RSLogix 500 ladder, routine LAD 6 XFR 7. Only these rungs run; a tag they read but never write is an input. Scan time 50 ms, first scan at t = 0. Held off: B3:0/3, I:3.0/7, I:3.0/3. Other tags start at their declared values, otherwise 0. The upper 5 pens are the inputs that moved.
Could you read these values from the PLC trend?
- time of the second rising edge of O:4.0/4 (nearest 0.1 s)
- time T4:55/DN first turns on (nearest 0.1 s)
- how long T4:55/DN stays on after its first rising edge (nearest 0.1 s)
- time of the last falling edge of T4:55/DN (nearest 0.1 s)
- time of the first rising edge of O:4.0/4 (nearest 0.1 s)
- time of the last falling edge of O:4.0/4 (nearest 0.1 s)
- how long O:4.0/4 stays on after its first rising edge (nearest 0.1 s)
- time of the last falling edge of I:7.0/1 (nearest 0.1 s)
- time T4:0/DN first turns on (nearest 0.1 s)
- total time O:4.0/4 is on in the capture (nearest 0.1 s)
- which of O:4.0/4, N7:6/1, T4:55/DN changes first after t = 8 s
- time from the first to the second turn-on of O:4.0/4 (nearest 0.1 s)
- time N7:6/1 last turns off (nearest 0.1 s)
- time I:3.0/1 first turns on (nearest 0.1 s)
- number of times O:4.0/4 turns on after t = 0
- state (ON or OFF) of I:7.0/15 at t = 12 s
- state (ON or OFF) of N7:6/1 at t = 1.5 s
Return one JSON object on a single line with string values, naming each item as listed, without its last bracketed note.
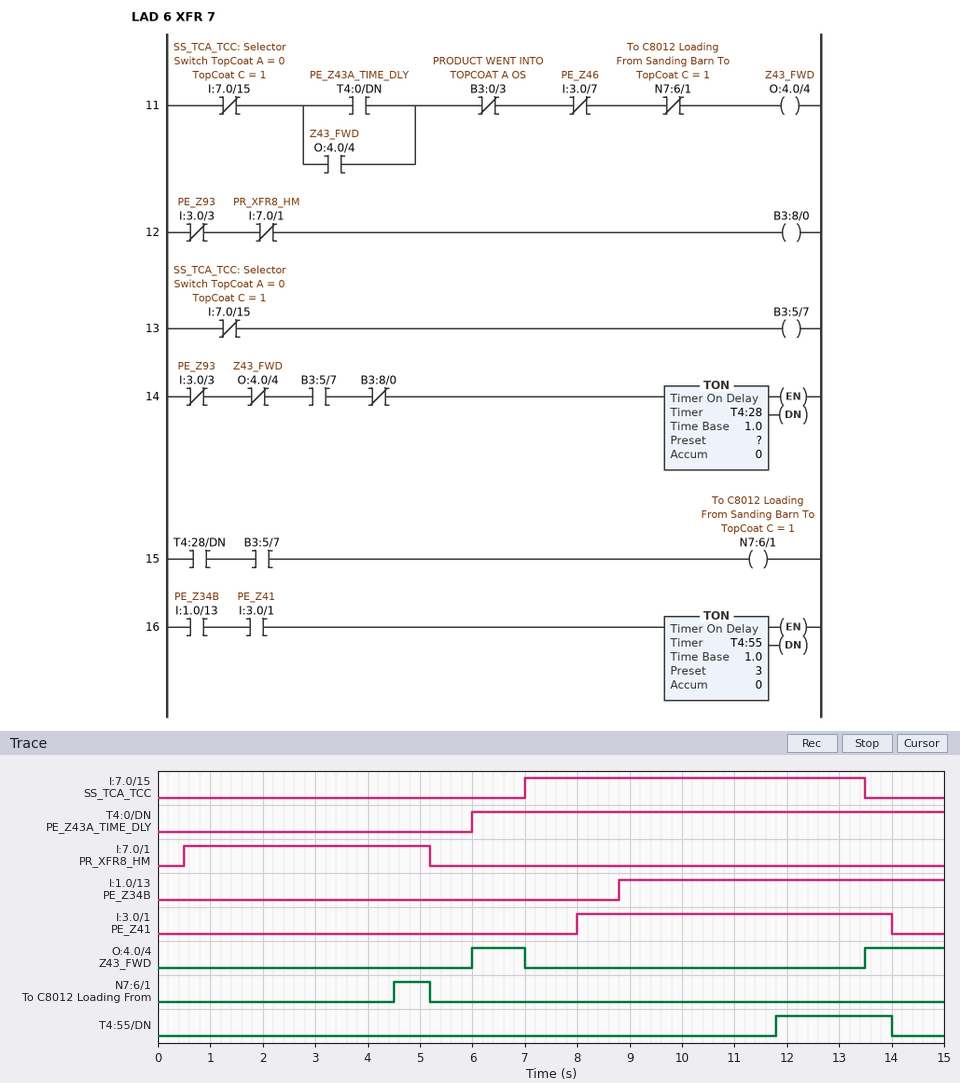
{"time of the second rising edge of O:4.0/4": "13.5 s", "time T4:55/DN first turns on": "11.8 s", "how long T4:55/DN stays on after its first rising edge": "2.2 s", "time of the last falling edge of T4:55/DN": "14.0 s", "time of the first rising edge of O:4.0/4": "6.0 s", "time of the last falling edge of O:4.0/4": "7.0 s", "how long O:4.0/4 stays on after its first rising edge": "1.0 s", "time of the last falling edge of I:7.0/1": "5.2 s", "time T4:0/DN first turns on": "6.0 s", "total time O:4.0/4 is on in the capture": "2.5 s", "which of O:4.0/4, N7:6/1, T4:55/DN changes first after t = 8 s": "T4:55/DN", "time from the first to the second turn-on of O:4.0/4": "7.5 s", "time N7:6/1 last turns off": "5.2 s", "time I:3.0/1 first turns on": "8.0 s", "number of times O:4.0/4 turns on after t = 0": "2", "state (ON or OFF) of I:7.0/15 at t = 12 s": "ON", "state (ON or OFF) of N7:6/1 at t = 1.5 s": "OFF"}
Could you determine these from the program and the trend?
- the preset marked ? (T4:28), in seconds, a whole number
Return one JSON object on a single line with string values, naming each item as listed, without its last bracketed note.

{"the preset marked ? (T4:28), in seconds, a whole number": "4 s"}
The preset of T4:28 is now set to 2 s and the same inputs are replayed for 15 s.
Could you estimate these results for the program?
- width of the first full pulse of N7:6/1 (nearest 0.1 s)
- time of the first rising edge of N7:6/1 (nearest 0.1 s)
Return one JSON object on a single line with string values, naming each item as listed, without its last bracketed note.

{"width of the first full pulse of N7:6/1": "2.7 s", "time of the first rising edge of N7:6/1": "2.5 s"}
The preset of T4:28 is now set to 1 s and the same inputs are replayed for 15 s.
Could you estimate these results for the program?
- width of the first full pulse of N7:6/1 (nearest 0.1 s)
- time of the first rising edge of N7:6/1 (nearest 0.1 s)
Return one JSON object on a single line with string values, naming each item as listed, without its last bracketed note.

{"width of the first full pulse of N7:6/1": "3.7 s", "time of the first rising edge of N7:6/1": "1.5 s"}
